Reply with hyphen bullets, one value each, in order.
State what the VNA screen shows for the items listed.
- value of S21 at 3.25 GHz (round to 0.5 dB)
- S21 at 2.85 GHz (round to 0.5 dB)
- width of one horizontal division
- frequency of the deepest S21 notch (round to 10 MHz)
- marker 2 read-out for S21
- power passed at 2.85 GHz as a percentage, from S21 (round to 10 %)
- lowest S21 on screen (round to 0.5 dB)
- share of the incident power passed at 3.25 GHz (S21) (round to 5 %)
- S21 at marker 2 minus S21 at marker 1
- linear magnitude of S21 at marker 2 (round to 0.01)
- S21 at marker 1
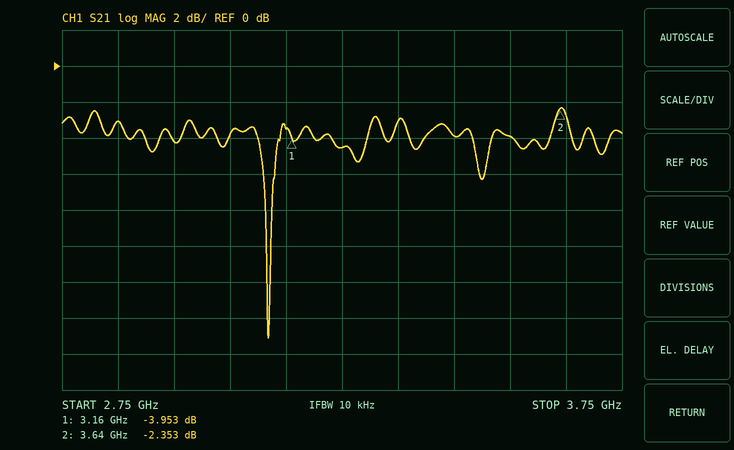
- -4.5 dB
- -3.0 dB
- 100 MHz
- 3.12 GHz
- -2.353 dB
- 50 %
- -15.0 dB
- 35 %
- 1.600 dB
- 0.76
- -3.953 dB
